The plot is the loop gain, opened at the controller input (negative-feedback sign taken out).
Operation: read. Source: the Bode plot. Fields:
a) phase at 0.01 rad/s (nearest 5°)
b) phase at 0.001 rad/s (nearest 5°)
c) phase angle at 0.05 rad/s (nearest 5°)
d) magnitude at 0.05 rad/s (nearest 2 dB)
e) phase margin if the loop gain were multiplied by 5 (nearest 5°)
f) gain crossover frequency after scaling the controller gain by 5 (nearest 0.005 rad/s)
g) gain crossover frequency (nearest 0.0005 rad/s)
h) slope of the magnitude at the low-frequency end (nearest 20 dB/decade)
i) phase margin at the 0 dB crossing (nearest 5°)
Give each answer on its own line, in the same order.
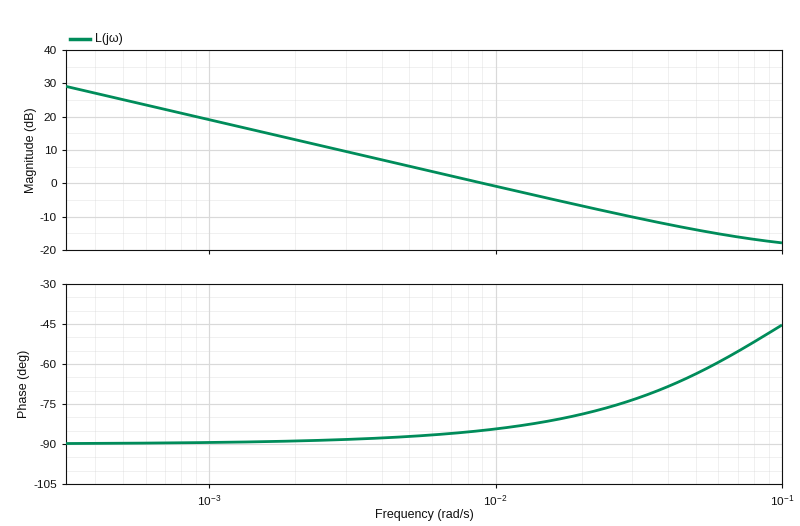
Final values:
-85°
-90°
-65°
-14 dB
115°
0.050 rad/s
0.0090 rad/s
-20 dB/decade
95°
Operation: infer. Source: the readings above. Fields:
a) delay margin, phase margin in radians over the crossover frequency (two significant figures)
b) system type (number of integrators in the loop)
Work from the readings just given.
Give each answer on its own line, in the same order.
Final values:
180 s
1
